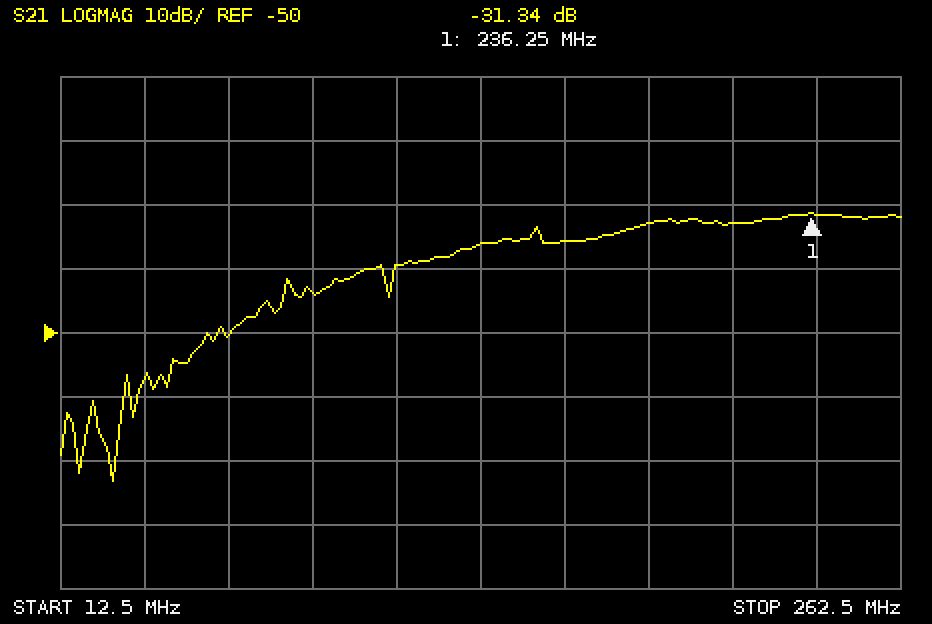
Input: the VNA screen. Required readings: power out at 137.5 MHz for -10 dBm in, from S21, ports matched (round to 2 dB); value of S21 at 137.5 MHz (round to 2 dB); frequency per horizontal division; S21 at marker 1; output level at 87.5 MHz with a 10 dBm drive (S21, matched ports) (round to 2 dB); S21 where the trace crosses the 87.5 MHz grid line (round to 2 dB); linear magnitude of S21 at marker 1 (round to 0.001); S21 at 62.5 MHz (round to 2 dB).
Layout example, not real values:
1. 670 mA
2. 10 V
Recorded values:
1. -46 dBm
2. -36 dB
3. 25 MHz
4. -31.34 dB
5. -34 dBm
6. -44 dB
7. 0.027
8. -50 dB
